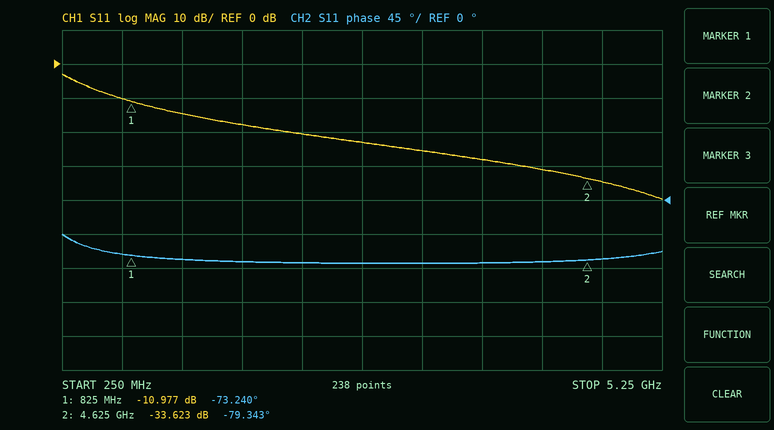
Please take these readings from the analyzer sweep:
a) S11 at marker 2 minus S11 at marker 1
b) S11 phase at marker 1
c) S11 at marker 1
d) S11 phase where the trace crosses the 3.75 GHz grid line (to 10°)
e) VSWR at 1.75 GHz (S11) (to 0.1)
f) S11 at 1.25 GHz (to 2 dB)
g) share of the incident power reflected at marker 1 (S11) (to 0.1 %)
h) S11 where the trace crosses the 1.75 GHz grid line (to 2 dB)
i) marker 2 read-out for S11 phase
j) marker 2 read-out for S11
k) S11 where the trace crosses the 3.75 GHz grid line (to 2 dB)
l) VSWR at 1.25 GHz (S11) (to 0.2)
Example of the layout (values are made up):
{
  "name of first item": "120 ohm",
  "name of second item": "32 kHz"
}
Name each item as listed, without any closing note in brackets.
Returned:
{
  "S11 at marker 2 minus S11 at marker 1": "-22.646 dB",
  "S11 phase at marker 1": "-73.240°",
  "S11 at marker 1": "-10.977 dB",
  "S11 phase where the trace crosses the 3.75 GHz grid line": "-80°",
  "VSWR at 1.75 GHz (S11)": "1.3",
  "S11 at 1.25 GHz": "-14 dB",
  "share of the incident power reflected at marker 1 (S11)": "8.0 %",
  "S11 where the trace crosses the 1.75 GHz grid line": "-18 dB",
  "marker 2 read-out for S11 phase": "-79.343°",
  "marker 2 read-out for S11": "-33.623 dB",
  "S11 where the trace crosses the 3.75 GHz grid line": "-28 dB",
  "VSWR at 1.25 GHz (S11)": "1.4"
}
